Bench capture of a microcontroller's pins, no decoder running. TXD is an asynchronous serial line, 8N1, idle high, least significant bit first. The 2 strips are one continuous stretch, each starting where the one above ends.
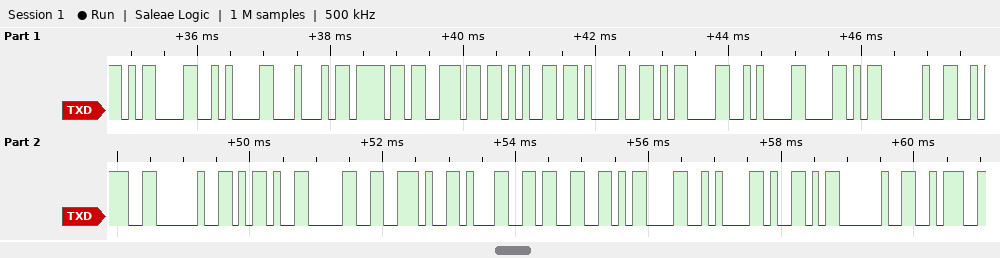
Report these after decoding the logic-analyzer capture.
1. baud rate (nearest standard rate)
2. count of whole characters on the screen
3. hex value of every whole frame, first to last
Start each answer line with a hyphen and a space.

- 9600 baud
- 23
- 0D 0A 44 6F 6E 65 21 0D 0A 58 20 3A 20 2D 30 2E 31 33 0D 0A 59 20 3A
